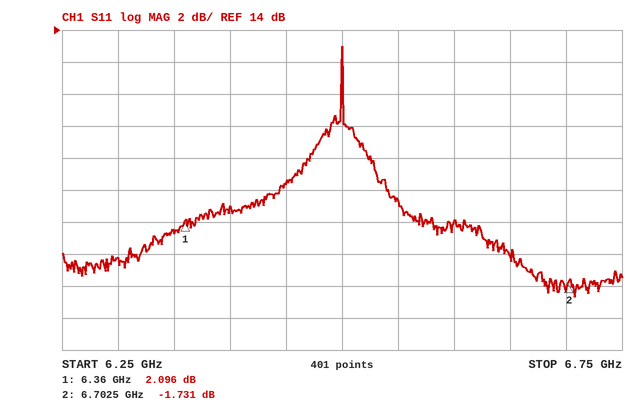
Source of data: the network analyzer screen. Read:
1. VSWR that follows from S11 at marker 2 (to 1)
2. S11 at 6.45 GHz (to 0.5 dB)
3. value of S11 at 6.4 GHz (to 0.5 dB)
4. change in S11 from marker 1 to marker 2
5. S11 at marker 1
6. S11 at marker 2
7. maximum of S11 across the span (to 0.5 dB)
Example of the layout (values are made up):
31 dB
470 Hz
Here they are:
10
4.5 dB
3.0 dB
-3.827 dB
2.096 dB
-1.731 dB
13.0 dB
